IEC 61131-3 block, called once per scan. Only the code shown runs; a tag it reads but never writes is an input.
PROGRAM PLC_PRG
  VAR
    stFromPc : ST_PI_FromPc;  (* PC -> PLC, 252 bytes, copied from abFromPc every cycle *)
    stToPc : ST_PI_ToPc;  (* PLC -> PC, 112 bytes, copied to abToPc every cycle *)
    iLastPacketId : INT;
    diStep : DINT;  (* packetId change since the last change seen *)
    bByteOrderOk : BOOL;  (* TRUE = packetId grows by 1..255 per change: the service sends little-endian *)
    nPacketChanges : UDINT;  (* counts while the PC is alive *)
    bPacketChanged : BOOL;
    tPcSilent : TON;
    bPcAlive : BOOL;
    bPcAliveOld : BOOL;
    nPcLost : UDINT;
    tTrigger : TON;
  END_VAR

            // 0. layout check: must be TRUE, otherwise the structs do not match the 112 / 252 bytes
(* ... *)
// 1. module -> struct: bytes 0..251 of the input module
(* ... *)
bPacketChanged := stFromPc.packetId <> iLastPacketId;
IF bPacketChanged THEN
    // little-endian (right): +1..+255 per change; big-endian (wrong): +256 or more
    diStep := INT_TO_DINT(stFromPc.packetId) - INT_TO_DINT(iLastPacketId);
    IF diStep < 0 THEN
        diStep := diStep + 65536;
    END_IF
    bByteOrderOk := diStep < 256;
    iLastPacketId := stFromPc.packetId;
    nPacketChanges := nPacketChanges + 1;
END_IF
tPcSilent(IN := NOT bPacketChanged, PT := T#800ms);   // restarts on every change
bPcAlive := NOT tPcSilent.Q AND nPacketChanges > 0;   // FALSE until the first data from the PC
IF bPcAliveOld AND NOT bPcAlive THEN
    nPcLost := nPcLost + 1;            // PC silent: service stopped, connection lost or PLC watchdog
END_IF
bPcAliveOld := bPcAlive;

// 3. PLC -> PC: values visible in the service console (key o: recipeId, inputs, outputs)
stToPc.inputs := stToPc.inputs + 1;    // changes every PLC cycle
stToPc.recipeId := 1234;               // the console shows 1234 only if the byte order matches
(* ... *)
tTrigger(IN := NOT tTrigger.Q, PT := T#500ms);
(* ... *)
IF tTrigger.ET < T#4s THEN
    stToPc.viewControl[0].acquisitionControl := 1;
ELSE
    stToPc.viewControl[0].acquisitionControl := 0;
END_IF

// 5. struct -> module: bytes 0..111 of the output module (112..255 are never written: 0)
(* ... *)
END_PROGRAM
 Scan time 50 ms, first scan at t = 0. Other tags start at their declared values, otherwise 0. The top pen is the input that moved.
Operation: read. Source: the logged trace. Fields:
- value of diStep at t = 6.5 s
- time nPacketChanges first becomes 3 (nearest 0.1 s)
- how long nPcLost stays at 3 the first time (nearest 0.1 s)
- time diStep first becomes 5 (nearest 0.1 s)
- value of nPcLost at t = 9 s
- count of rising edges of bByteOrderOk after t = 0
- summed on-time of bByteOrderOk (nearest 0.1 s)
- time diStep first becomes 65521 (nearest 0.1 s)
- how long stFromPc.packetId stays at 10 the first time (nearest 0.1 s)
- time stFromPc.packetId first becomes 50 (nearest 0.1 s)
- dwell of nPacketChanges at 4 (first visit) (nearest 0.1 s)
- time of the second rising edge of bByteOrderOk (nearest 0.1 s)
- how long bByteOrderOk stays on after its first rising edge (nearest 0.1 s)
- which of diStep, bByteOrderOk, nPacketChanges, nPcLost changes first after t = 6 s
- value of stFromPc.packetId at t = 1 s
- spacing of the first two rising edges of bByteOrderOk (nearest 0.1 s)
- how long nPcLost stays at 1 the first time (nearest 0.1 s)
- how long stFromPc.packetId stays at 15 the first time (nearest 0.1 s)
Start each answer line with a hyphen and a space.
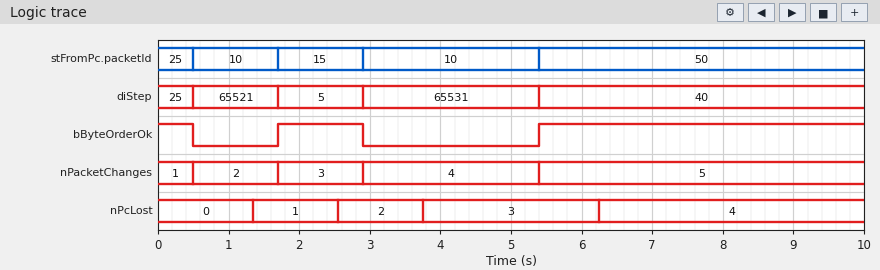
- 40
- 1.7 s
- 2.5 s
- 1.7 s
- 4
- 2
- 6.3 s
- 0.5 s
- 1.2 s
- 5.4 s
- 2.5 s
- 5.4 s
- 1.2 s
- nPcLost
- 10
- 3.7 s
- 1.2 s
- 1.2 s
